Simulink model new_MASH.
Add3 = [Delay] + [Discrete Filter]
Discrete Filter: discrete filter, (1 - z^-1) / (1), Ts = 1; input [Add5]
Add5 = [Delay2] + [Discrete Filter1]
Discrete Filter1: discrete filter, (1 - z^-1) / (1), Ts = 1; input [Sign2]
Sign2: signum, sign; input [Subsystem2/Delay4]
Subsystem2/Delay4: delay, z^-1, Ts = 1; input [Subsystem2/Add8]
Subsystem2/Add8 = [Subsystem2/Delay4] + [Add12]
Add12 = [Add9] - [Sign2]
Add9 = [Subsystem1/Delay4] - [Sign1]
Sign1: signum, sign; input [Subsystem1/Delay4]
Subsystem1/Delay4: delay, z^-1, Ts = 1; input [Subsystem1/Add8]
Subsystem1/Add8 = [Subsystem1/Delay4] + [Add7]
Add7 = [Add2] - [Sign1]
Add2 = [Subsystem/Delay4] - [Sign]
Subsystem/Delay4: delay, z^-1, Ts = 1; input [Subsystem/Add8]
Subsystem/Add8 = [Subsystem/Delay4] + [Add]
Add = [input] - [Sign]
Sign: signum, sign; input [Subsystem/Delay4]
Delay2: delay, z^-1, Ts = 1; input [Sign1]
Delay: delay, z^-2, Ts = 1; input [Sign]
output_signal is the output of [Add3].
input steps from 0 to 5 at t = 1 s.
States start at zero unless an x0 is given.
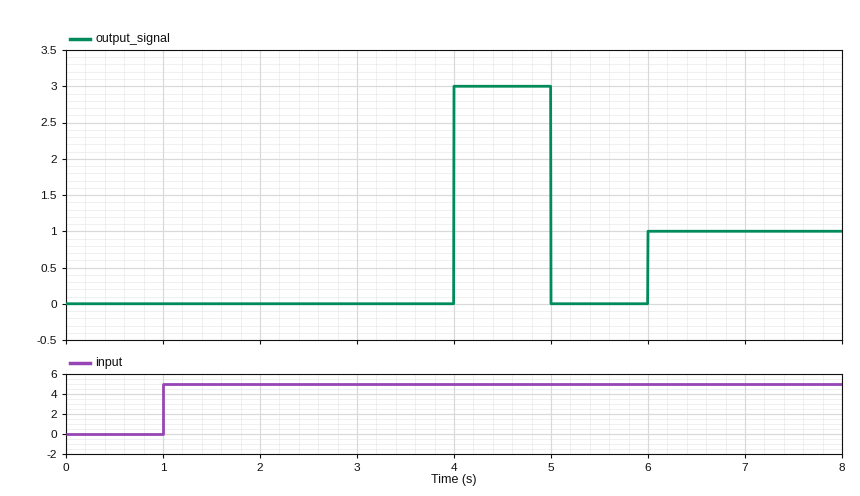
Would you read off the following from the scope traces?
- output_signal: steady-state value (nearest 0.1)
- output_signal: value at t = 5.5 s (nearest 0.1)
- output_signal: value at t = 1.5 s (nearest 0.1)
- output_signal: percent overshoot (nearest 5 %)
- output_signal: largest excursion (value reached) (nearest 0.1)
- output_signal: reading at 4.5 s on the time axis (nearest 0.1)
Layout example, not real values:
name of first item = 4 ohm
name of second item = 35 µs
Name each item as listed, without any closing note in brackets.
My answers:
output_signal: steady-state value = 1.0
output_signal: value at t = 5.5 s = 0.0
output_signal: value at t = 1.5 s = 0.0
output_signal: percent overshoot = 200 %
output_signal: largest excursion (value reached) = 3.0
output_signal: reading at 4.5 s on the time axis = 3.0
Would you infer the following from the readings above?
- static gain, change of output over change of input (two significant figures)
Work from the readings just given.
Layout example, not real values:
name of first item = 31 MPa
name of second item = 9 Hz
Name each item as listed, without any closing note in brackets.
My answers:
static gain, change of output over change of input = 0.20
